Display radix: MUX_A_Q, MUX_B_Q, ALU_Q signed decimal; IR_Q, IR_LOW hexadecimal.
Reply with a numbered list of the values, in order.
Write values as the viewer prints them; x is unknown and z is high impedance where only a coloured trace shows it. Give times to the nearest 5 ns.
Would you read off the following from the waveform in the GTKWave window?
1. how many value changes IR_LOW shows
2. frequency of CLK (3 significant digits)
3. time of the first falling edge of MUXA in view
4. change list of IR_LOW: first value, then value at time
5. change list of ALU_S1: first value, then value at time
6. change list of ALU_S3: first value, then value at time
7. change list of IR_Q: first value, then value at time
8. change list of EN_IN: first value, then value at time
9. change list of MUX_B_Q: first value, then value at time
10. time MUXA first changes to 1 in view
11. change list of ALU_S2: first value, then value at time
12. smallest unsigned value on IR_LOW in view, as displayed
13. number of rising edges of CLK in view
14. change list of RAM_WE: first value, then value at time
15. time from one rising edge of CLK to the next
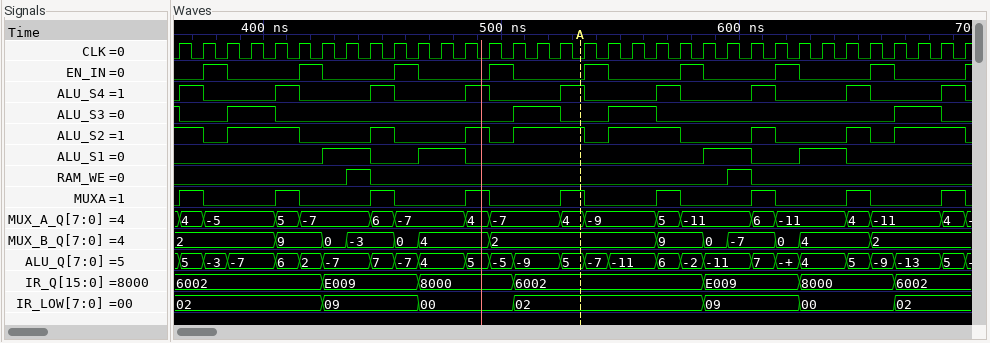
1. 6
2. 100 MHz
3. 375 ns
4. 02, 09 at 425 ns, 00 at 465 ns, 02 at 505 ns, 09 at 585 ns, 00 at 625 ns, 02 at 665 ns
5. 0, 1 at 425 ns, 0 at 445 ns, 1 at 465 ns, 0 at 485 ns, 1 at 585 ns, 0 at 605 ns, 1 at 625 ns, 0 at 645 ns
6. 1, 0 at 365 ns, 1 at 385 ns, 0 at 405 ns, 1 at 505 ns, 0 at 525 ns, 1 at 545 ns, 0 at 565 ns, 1 at 665 ns, 0 at 685 ns
7. 6002, E009 at 425 ns, 8000 at 465 ns, 6002 at 505 ns, E009 at 585 ns, 8000 at 625 ns, 6002 at 665 ns
8. 0, 1 at 375 ns, 0 at 385 ns, 1 at 415 ns, 0 at 425 ns, 1 at 455 ns, 0 at 465 ns, 1 at 495 ns, 0 at 505 ns, 1 at 535 ns, 0 at 545 ns, 1 at 575 ns, 0 at 585 ns, 1 at 615 ns, 0 at 625 ns, 1 at 655 ns, 0 at 665 ns, 1 at 695 ns
9. 2, 9 at 405 ns, 0 at 425 ns, -3 at 435 ns, 0 at 455 ns, 4 at 465 ns, 2 at 495 ns, 9 at 565 ns, 0 at 585 ns, -7 at 595 ns, 0 at 615 ns, 4 at 625 ns, 2 at 655 ns
10. 365 ns
11. 1, 0 at 375 ns, 1 at 385 ns, 0 at 415 ns, 1 at 445 ns, 0 at 455 ns, 1 at 485 ns, 0 at 495 ns, 1 at 505 ns, 0 at 535 ns, 1 at 545 ns, 0 at 575 ns, 1 at 605 ns, 0 at 615 ns, 1 at 645 ns, 0 at 655 ns, 1 at 665 ns, 0 at 695 ns
12. 00
13. 34
14. 0, 1 at 435 ns, 0 at 445 ns, 1 at 595 ns, 0 at 605 ns
15. 10 ns
